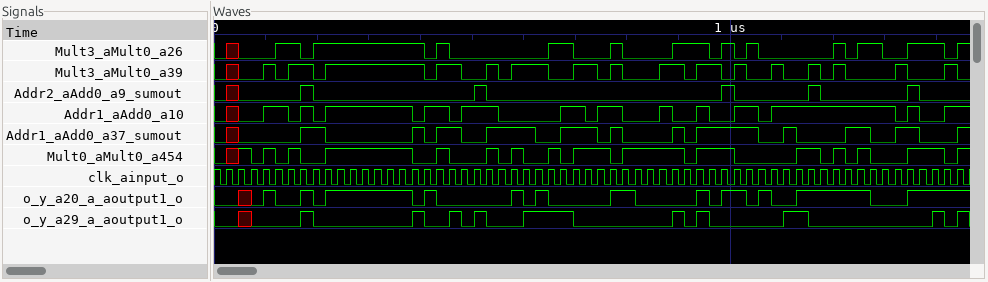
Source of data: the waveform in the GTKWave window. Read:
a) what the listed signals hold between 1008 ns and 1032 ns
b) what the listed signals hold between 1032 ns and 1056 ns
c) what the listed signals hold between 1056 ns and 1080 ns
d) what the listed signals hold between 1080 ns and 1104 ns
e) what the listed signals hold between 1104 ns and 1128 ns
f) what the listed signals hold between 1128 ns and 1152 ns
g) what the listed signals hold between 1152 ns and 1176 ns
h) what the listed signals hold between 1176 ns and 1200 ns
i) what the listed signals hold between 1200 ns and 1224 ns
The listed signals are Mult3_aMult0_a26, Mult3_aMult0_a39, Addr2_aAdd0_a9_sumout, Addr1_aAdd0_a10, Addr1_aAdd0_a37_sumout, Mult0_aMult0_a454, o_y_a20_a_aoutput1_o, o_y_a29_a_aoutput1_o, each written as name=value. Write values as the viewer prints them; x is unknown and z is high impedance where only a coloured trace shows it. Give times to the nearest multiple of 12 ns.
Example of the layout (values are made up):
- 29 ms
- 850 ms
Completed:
- Mult3_aMult0_a26=0, Mult3_aMult0_a39=1, Addr2_aAdd0_a9_sumout=0, Addr1_aAdd0_a10=1, Addr1_aAdd0_a37_sumout=1, Mult0_aMult0_a454=0, o_y_a20_a_aoutput1_o=1, o_y_a29_a_aoutput1_o=0
- Mult3_aMult0_a26=1, Mult3_aMult0_a39=0, Addr2_aAdd0_a9_sumout=0, Addr1_aAdd0_a10=1, Addr1_aAdd0_a37_sumout=1, Mult0_aMult0_a454=0, o_y_a20_a_aoutput1_o=0, o_y_a29_a_aoutput1_o=0
- Mult3_aMult0_a26=0, Mult3_aMult0_a39=0, Addr2_aAdd0_a9_sumout=0, Addr1_aAdd0_a10=0, Addr1_aAdd0_a37_sumout=0, Mult0_aMult0_a454=0, o_y_a20_a_aoutput1_o=1, o_y_a29_a_aoutput1_o=0
- Mult3_aMult0_a26=0, Mult3_aMult0_a39=1, Addr2_aAdd0_a9_sumout=0, Addr1_aAdd0_a10=1, Addr1_aAdd0_a37_sumout=0, Mult0_aMult0_a454=0, o_y_a20_a_aoutput1_o=0, o_y_a29_a_aoutput1_o=0
- Mult3_aMult0_a26=0, Mult3_aMult0_a39=0, Addr2_aAdd0_a9_sumout=0, Addr1_aAdd0_a10=1, Addr1_aAdd0_a37_sumout=1, Mult0_aMult0_a454=0, o_y_a20_a_aoutput1_o=0, o_y_a29_a_aoutput1_o=1
- Mult3_aMult0_a26=0, Mult3_aMult0_a39=0, Addr2_aAdd0_a9_sumout=0, Addr1_aAdd0_a10=1, Addr1_aAdd0_a37_sumout=0, Mult0_aMult0_a454=1, o_y_a20_a_aoutput1_o=1, o_y_a29_a_aoutput1_o=1
- Mult3_aMult0_a26=0, Mult3_aMult0_a39=1, Addr2_aAdd0_a9_sumout=1, Addr1_aAdd0_a10=1, Addr1_aAdd0_a37_sumout=0, Mult0_aMult0_a454=1, o_y_a20_a_aoutput1_o=1, o_y_a29_a_aoutput1_o=0
- Mult3_aMult0_a26=0, Mult3_aMult0_a39=0, Addr2_aAdd0_a9_sumout=0, Addr1_aAdd0_a10=1, Addr1_aAdd0_a37_sumout=0, Mult0_aMult0_a454=0, o_y_a20_a_aoutput1_o=1, o_y_a29_a_aoutput1_o=0
- Mult3_aMult0_a26=1, Mult3_aMult0_a39=1, Addr2_aAdd0_a9_sumout=0, Addr1_aAdd0_a10=1, Addr1_aAdd0_a37_sumout=0, Mult0_aMult0_a454=1, o_y_a20_a_aoutput1_o=1, o_y_a29_a_aoutput1_o=0
